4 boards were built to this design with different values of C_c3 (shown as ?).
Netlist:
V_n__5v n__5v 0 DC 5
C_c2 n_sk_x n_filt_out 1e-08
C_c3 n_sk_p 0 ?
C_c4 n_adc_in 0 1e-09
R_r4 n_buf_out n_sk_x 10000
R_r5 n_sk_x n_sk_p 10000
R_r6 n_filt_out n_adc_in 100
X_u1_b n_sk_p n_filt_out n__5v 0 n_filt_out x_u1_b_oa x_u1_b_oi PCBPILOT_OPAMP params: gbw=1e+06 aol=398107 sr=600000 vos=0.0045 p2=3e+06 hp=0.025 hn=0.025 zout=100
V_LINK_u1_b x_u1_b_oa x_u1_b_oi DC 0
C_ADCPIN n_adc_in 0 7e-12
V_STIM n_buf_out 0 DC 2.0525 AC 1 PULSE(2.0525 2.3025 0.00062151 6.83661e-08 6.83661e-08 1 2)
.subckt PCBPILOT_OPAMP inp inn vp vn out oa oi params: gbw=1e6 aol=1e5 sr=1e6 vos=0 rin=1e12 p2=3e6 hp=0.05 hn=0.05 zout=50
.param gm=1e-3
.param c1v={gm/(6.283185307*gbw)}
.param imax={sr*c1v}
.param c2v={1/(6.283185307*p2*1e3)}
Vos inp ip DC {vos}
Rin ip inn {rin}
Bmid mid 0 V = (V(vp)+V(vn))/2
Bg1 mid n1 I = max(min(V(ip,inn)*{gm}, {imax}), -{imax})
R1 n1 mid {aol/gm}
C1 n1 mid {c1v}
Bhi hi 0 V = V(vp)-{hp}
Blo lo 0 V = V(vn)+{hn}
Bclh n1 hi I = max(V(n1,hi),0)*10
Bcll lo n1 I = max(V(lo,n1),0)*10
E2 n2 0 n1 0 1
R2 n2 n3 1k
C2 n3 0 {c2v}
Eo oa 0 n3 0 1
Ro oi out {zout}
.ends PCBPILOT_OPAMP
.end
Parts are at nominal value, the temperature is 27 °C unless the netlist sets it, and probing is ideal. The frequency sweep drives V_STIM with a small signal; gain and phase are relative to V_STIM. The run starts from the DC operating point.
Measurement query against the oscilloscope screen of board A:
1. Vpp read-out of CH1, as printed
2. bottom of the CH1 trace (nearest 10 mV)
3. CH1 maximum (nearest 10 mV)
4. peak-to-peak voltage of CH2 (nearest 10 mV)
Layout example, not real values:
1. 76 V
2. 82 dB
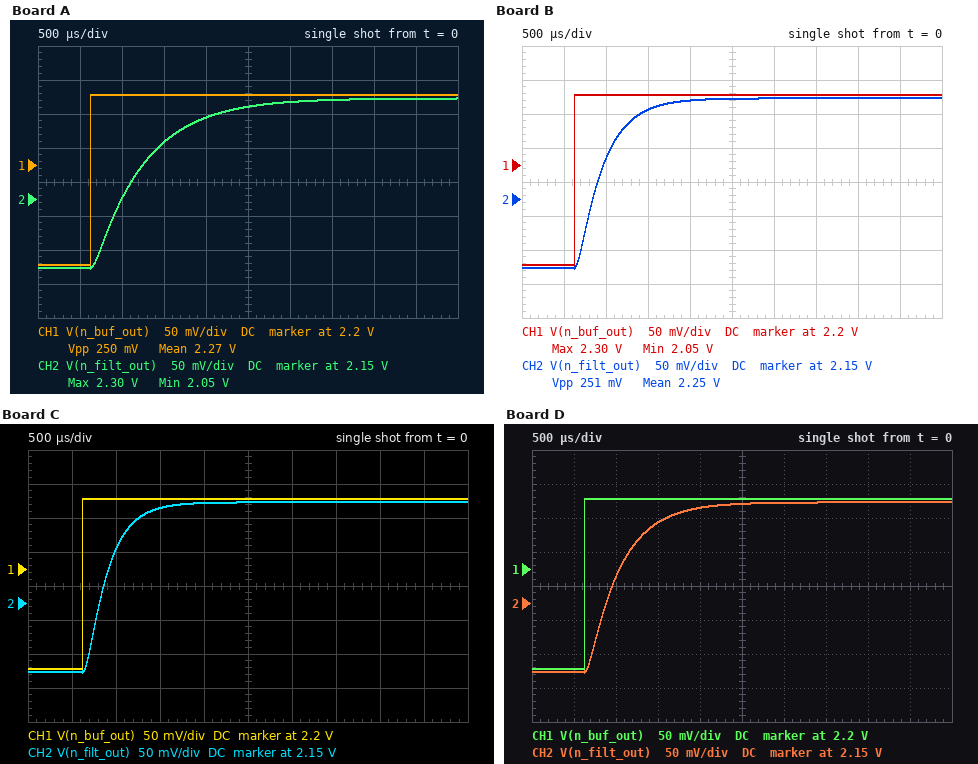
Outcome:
1. 250 mV
2. 2.05 V
3. 2.30 V
4. 250 mV
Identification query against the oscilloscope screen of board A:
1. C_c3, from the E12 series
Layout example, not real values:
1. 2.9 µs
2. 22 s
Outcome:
1. 33 nF
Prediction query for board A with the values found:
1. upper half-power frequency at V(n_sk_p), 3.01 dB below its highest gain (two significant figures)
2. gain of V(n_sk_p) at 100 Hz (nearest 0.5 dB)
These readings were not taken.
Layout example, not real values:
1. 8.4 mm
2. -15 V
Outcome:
1. 260 Hz
2. -0.5 dB
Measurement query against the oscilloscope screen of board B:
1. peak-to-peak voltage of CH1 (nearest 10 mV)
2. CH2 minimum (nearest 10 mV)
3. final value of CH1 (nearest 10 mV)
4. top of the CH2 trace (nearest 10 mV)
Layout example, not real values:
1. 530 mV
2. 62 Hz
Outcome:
1. 250 mV
2. 2.05 V
3. 2.30 V
4. 2.30 V
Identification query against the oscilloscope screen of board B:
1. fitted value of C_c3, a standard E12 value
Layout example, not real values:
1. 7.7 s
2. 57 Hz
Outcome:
1. 18 nF
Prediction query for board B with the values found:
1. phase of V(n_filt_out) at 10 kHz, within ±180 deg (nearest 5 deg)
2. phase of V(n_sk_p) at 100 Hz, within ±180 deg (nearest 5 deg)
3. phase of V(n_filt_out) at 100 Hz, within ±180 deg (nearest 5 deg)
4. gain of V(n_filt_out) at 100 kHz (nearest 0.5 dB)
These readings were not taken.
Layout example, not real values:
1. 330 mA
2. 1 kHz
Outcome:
1. -165 deg
2. -15 deg
3. -15 deg
4. -60.0 dB
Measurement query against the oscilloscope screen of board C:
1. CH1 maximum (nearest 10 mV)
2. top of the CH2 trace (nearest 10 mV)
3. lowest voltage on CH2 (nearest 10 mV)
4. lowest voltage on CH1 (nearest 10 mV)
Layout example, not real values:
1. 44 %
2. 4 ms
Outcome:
1. 2.30 V
2. 2.30 V
3. 2.05 V
4. 2.05 V
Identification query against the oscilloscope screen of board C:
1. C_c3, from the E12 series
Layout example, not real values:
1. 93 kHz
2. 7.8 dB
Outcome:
1. 15 nF
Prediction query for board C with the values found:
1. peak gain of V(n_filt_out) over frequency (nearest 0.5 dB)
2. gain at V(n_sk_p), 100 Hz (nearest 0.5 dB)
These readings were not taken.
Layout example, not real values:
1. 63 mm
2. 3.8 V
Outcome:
1. 0 dB
2. 0 dB
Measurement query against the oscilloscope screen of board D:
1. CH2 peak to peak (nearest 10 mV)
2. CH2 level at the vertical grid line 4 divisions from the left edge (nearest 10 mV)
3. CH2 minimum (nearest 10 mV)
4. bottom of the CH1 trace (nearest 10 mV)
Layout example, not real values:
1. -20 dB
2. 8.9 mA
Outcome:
1. 250 mV
2. 2.29 V
3. 2.05 V
4. 2.05 V
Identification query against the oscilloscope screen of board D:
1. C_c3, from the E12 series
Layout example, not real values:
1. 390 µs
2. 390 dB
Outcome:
1. 22 nF
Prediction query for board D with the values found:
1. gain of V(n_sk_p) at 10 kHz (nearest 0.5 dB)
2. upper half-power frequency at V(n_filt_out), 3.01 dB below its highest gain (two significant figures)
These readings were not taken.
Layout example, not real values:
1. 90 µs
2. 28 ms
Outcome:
1. -39.0 dB
2. 410 Hz
